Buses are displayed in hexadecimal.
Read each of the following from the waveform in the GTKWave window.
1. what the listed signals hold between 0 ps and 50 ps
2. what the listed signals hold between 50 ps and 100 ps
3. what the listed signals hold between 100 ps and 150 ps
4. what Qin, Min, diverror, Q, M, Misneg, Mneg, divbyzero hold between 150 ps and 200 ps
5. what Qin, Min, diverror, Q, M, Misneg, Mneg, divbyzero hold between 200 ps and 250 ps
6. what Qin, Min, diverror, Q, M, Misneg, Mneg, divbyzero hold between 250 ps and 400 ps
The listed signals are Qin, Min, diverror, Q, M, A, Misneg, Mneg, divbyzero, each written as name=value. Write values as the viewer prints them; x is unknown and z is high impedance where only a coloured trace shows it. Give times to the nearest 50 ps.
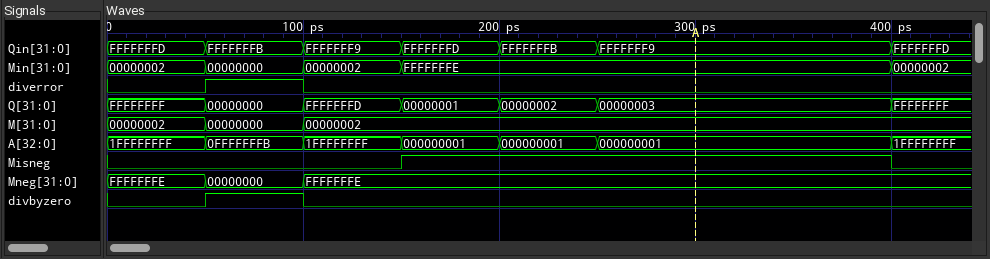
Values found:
Qin=FFFFFFFD, Min=00000002, diverror=0, Q=FFFFFFFF, M=00000002, A=1FFFFFFFF, Misneg=0, Mneg=FFFFFFFE, divbyzero=0
Qin=FFFFFFFB, Min=00000000, diverror=1, Q=00000000, M=00000000, A=0FFFFFFFB, Misneg=0, Mneg=00000000, divbyzero=1
Qin=FFFFFFF9, Min=00000002, diverror=0, Q=FFFFFFFD, M=00000002, A=1FFFFFFFF, Misneg=0, Mneg=FFFFFFFE, divbyzero=0
Qin=FFFFFFFD, Min=FFFFFFFE, diverror=0, Q=00000001, M=00000002, Misneg=1, Mneg=FFFFFFFE, divbyzero=0
Qin=FFFFFFFB, Min=FFFFFFFE, diverror=0, Q=00000002, M=00000002, Misneg=1, Mneg=FFFFFFFE, divbyzero=0
Qin=FFFFFFF9, Min=FFFFFFFE, diverror=0, Q=00000003, M=00000002, Misneg=1, Mneg=FFFFFFFE, divbyzero=0
